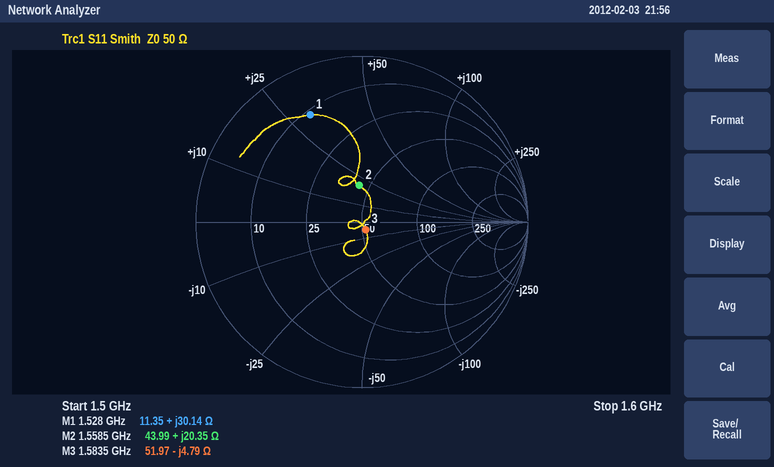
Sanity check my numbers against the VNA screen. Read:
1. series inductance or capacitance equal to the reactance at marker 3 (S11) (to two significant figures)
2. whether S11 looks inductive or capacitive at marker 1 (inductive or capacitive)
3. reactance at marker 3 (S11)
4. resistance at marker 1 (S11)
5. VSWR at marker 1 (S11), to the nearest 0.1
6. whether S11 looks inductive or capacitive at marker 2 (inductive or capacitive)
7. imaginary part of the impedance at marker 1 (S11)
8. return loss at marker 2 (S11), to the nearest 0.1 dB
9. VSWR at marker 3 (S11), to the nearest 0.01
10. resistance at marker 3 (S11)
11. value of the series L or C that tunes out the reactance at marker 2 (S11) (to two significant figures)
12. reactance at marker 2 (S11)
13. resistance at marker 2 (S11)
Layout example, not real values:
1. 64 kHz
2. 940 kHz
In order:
1. 21 pF
2. inductive
3. -4.79 Ω
4. 11.35 Ω
5. 6.1
6. inductive
7. +30.14 Ω
8. 13.1 dB
9. 1.11
10. 51.97 Ω
11. 5.0 pF
12. +20.35 Ω
13. 43.99 Ω
